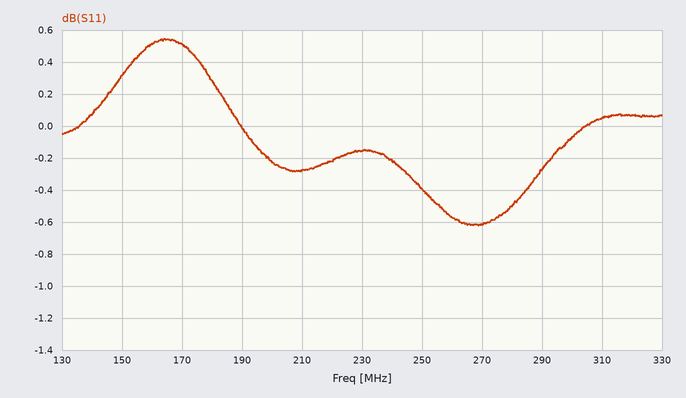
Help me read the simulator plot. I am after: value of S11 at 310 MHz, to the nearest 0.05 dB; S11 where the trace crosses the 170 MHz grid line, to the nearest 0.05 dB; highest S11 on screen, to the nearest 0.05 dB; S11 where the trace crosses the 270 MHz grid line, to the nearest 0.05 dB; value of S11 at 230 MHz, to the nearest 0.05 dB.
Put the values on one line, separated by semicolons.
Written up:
0.05 dB; 0.50 dB; 0.55 dB; -0.60 dB; -0.15 dB
